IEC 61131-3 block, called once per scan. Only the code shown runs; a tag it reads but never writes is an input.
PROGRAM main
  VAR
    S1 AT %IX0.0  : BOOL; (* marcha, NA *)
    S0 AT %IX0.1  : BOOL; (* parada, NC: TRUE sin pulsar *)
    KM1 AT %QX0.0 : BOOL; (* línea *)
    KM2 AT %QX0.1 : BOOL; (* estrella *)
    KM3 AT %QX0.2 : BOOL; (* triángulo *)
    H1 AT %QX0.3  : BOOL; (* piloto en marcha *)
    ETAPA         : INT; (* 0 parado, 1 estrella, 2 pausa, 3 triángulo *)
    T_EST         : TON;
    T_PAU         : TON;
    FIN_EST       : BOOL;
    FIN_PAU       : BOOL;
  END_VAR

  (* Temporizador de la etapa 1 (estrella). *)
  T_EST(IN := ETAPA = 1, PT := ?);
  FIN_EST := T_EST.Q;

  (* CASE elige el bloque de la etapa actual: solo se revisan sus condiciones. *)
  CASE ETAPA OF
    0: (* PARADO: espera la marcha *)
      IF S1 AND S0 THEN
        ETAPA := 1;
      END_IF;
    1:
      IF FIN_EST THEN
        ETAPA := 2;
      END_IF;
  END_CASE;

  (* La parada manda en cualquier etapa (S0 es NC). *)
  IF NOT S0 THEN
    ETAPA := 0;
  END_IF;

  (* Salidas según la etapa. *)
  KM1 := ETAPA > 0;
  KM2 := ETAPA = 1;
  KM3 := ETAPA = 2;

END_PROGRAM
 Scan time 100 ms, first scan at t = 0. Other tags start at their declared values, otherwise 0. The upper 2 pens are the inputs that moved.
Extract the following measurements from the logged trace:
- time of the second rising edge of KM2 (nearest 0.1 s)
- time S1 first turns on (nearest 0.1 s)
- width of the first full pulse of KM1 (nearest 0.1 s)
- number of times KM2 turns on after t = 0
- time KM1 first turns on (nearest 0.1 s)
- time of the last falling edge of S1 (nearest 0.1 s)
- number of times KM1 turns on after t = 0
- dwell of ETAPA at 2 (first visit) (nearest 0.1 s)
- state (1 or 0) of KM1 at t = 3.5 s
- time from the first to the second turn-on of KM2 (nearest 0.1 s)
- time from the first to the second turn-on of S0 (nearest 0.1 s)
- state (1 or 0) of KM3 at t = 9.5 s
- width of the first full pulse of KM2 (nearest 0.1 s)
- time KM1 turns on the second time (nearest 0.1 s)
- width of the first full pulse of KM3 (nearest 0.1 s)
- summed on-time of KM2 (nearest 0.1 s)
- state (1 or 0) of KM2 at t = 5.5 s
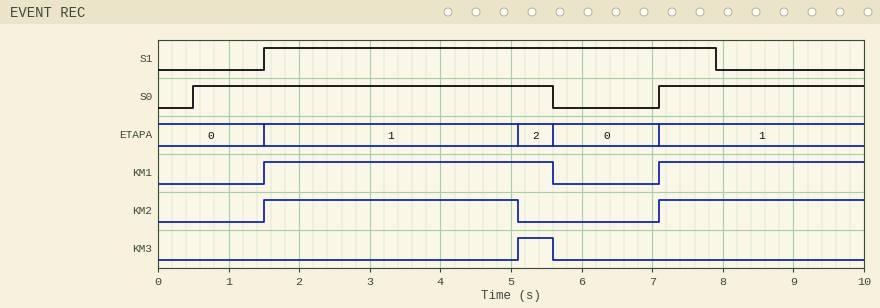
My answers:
7.1 s
1.5 s
4.1 s
2
1.5 s
7.9 s
2
0.5 s
1
5.6 s
6.6 s
0
3.6 s
7.1 s
0.5 s
6.5 s
0
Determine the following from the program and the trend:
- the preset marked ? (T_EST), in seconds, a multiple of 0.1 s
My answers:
3.5 s
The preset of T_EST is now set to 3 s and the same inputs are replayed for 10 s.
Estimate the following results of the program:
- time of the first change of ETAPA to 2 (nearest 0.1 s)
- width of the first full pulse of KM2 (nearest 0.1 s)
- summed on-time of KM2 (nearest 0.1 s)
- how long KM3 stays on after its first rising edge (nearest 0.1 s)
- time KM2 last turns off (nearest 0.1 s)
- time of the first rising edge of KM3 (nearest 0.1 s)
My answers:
4.6 s
3.1 s
6.0 s
1.0 s
4.6 s
4.6 s
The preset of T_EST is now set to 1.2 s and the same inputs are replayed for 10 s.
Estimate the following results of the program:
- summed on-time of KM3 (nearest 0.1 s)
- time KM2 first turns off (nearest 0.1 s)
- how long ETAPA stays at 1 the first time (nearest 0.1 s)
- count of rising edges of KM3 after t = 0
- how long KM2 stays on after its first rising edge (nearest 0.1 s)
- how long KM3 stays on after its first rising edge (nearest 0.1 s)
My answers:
4.4 s
2.8 s
1.3 s
2
1.3 s
2.8 s
